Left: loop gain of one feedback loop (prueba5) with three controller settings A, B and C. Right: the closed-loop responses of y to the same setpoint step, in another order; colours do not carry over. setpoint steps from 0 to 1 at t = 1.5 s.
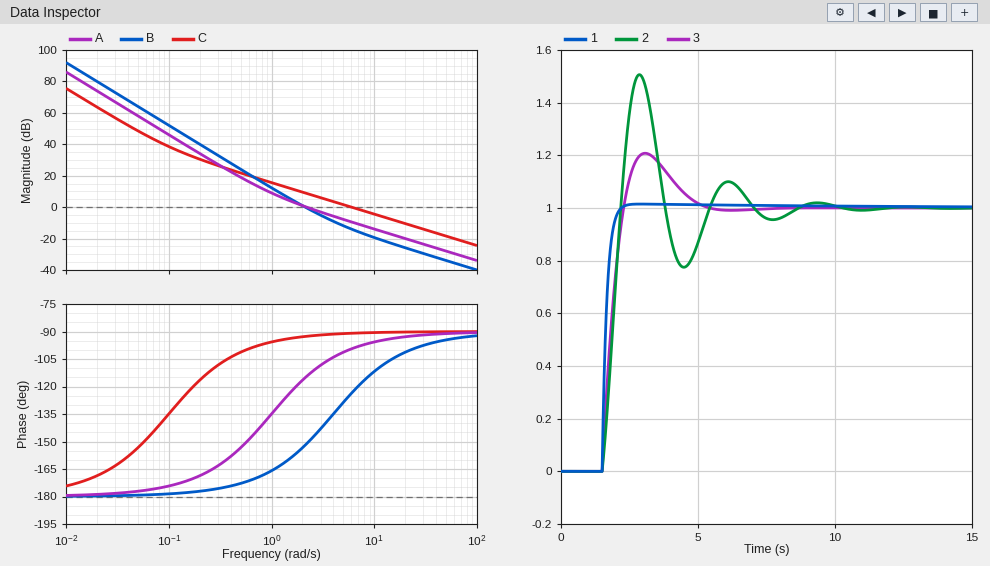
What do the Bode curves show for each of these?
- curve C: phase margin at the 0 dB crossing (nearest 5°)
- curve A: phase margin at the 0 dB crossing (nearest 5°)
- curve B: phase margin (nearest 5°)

90°
65°
30°
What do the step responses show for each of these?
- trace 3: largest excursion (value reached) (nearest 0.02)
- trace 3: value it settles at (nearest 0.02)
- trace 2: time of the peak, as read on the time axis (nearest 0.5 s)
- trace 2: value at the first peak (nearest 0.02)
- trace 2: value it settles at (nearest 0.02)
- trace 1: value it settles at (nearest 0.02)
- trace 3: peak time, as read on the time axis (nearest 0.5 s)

1.20
1.00
3.0 s
1.50
1.00
1.00
3.0 s
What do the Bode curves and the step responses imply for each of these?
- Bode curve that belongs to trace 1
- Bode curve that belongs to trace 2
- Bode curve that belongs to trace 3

C
B
A
